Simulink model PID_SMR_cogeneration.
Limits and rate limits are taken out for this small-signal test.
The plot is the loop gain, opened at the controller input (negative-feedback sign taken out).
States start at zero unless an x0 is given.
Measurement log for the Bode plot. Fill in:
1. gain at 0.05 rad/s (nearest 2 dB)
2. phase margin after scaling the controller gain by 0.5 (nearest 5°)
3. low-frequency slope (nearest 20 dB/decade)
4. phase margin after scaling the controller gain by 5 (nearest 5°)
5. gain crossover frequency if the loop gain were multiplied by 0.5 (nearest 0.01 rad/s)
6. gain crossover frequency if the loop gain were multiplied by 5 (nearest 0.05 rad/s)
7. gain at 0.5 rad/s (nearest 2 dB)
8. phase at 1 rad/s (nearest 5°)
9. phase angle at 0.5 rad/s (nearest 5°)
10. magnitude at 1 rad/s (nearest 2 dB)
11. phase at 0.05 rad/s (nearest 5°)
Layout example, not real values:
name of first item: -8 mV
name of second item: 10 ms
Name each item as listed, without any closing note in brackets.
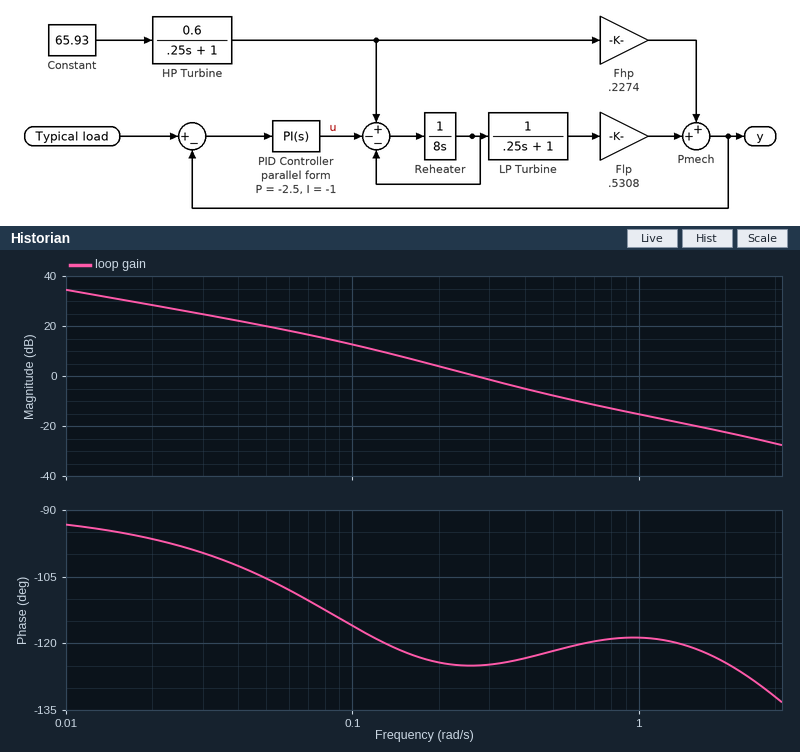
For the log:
gain at 0.05 rad/s: 20 dB
phase margin after scaling the controller gain by 0.5: 55°
low-frequency slope: -20 dB/decade
phase margin after scaling the controller gain by 5: 60°
gain crossover frequency if the loop gain were multiplied by 0.5: 0.17 rad/s
gain crossover frequency if the loop gain were multiplied by 5: 0.90 rad/s
gain at 0.5 rad/s: -8 dB
phase at 1 rad/s: -120°
phase angle at 0.5 rad/s: -120°
magnitude at 1 rad/s: -16 dB
phase at 0.05 rad/s: -105°
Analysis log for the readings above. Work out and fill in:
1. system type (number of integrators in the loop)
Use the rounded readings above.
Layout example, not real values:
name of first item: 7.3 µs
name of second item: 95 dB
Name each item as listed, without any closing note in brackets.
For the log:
system type: 1
